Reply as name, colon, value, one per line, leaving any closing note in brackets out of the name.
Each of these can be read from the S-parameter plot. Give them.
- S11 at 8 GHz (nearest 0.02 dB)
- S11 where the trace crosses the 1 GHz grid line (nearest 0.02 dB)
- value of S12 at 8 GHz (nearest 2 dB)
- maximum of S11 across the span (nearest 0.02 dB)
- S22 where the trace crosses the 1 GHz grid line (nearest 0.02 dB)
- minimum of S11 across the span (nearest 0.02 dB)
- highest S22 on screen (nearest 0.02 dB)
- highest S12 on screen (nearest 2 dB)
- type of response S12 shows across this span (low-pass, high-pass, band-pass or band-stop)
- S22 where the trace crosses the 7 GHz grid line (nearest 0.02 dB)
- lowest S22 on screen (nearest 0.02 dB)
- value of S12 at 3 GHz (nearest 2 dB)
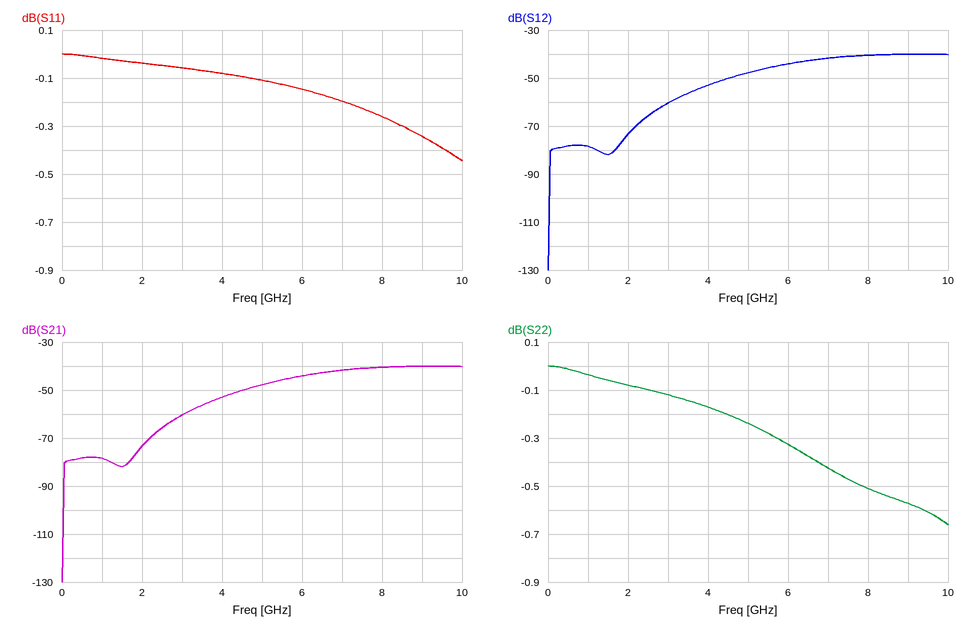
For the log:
S11 at 8 GHz: -0.26 dB
S11 where the trace crosses the 1 GHz grid line: -0.02 dB
value of S12 at 8 GHz: -40 dB
maximum of S11 across the span: 0.00 dB
S22 where the trace crosses the 1 GHz grid line: -0.04 dB
minimum of S11 across the span: -0.44 dB
highest S22 on screen: 0.00 dB
highest S12 on screen: -40 dB
type of response S12 shows across this span: high-pass
S22 where the trace crosses the 7 GHz grid line: -0.42 dB
lowest S22 on screen: -0.66 dB
value of S12 at 3 GHz: -60 dB
